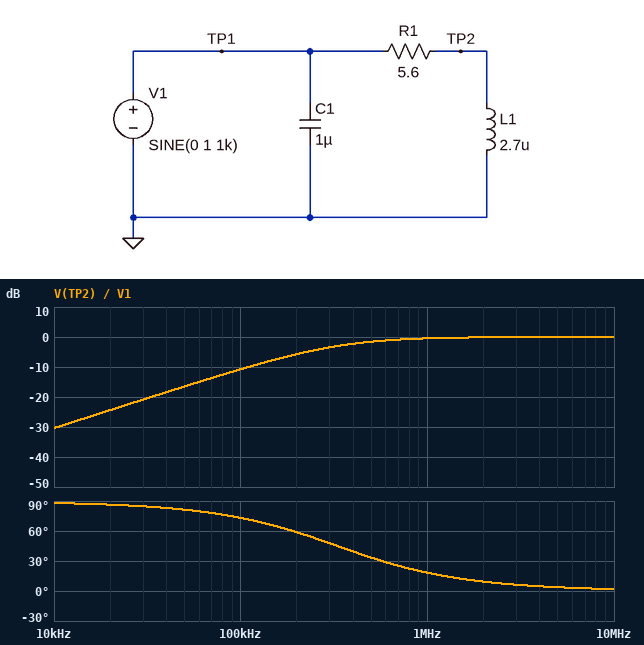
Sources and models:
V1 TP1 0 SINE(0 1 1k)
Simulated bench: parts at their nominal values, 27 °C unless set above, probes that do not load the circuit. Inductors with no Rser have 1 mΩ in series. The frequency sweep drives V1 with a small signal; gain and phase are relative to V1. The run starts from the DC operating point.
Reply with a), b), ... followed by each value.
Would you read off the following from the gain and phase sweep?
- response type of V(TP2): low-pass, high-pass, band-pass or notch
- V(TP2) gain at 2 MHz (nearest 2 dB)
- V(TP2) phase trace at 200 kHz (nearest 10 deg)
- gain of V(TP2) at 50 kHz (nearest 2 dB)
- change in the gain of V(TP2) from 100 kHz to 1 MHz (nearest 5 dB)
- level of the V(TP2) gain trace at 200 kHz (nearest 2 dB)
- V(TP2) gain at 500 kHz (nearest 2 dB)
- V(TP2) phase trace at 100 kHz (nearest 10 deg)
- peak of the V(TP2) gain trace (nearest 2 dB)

a) high-pass
b) 0 dB
c) 60 deg
d) -16 dB
e) 10 dB
f) -6 dB
g) -2 dB
h) 70 deg
i) 0 dB
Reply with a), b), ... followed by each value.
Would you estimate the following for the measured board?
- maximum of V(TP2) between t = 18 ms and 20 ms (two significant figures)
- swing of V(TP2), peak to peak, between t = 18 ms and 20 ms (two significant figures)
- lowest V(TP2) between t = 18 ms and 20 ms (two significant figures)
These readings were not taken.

a) 3.0 mV
b) 6.1 mV
c) -3.0 mV
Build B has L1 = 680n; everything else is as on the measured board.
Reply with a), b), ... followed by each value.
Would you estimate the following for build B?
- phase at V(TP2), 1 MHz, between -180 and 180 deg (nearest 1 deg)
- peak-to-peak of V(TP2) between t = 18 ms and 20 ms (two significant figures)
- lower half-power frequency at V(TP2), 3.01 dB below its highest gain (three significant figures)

a) 53 deg
b) 1.6 mV
c) 1.31 MHz
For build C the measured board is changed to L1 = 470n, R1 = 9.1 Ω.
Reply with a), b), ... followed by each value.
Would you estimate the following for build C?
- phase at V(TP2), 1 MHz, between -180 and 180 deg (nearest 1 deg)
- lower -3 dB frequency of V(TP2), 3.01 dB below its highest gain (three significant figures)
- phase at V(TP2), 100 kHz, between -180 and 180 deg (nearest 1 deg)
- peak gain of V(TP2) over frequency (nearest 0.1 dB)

a) 72 deg
b) 3.08 MHz
c) 88 deg
d) 0 dB
